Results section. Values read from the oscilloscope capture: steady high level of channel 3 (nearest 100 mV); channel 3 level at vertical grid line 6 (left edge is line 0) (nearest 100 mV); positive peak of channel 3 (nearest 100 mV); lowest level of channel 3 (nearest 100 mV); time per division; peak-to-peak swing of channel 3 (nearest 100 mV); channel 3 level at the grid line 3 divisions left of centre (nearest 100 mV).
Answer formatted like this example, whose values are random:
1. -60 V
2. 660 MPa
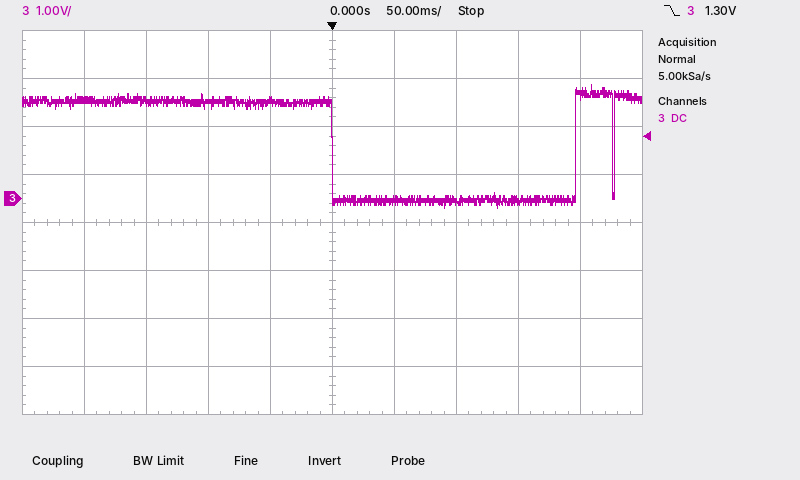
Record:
1. 2.0 V
2. 0.0 V
3. 2.4 V
4. -200 mV
5. 50 ms
6. 2.6 V
7. 2.0 V
